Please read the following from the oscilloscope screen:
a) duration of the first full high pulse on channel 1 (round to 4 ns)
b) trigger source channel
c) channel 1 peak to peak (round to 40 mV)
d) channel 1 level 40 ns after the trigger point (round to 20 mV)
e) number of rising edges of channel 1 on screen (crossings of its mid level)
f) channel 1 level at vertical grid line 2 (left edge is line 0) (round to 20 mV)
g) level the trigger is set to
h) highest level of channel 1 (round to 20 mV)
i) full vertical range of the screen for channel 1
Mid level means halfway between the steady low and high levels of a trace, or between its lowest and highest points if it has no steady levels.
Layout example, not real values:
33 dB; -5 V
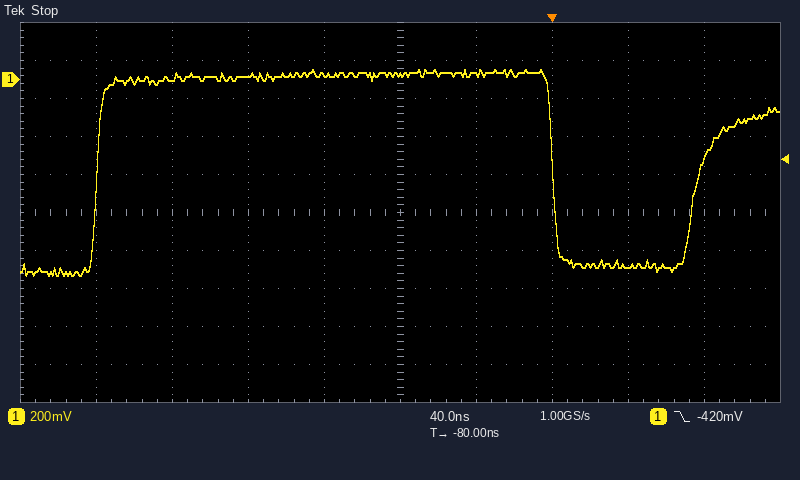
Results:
240 ns; channel 1; 1.08 V; -980 mV; 2; 20 mV; -420 mV; 60 mV; 2 V
